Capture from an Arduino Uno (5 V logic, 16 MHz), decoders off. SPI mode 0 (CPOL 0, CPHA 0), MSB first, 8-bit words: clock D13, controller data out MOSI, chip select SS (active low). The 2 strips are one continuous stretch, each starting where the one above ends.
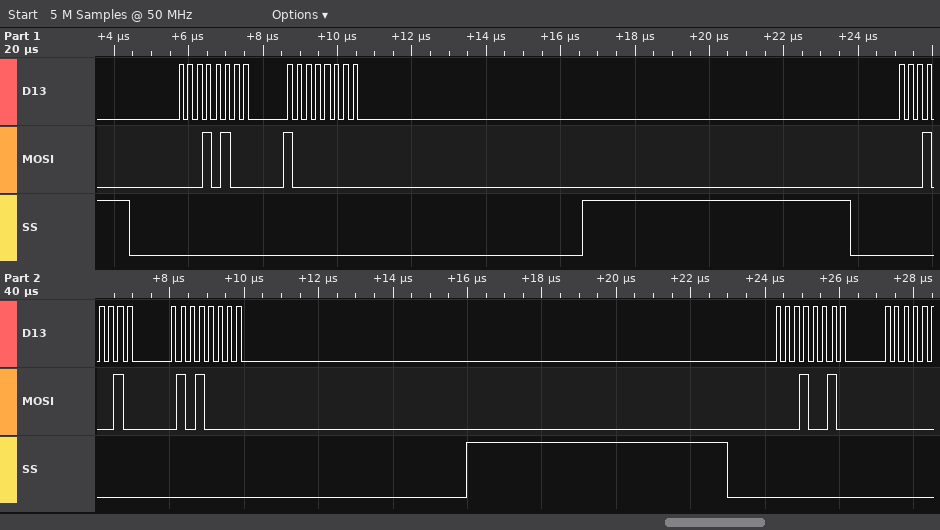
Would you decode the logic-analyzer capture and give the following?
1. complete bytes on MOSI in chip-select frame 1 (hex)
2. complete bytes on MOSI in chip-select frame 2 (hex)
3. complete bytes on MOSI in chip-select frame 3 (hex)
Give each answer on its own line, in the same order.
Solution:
14 80
12 50
12
